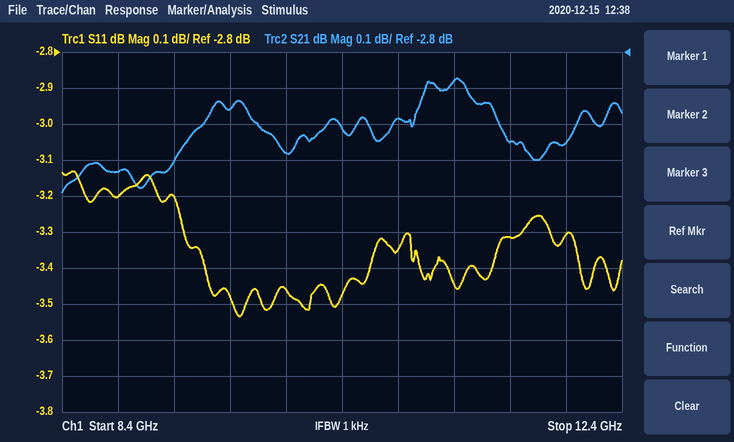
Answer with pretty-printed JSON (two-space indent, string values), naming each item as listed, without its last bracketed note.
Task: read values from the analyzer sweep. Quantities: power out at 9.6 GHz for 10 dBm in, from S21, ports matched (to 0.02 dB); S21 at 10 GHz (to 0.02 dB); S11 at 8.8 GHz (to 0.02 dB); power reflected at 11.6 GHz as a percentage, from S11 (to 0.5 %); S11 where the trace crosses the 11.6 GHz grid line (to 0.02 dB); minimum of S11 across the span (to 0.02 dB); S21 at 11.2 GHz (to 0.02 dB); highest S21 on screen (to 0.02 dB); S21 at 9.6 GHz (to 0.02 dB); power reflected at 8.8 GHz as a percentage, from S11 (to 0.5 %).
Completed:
{
  "power out at 9.6 GHz for 10 dBm in, from S21, ports matched": "7.04 dBm",
  "S21 at 10 GHz": "-3.08 dB",
  "S11 at 8.8 GHz": "-3.20 dB",
  "power reflected at 11.6 GHz as a percentage, from S11": "46.5 %",
  "S11 where the trace crosses the 11.6 GHz grid line": "-3.32 dB",
  "minimum of S11 across the span": "-3.54 dB",
  "S21 at 11.2 GHz": "-2.88 dB",
  "highest S21 on screen": "-2.88 dB",
  "S21 at 9.6 GHz": "-2.96 dB",
  "power reflected at 8.8 GHz as a percentage, from S11": "48.0 %"
}
